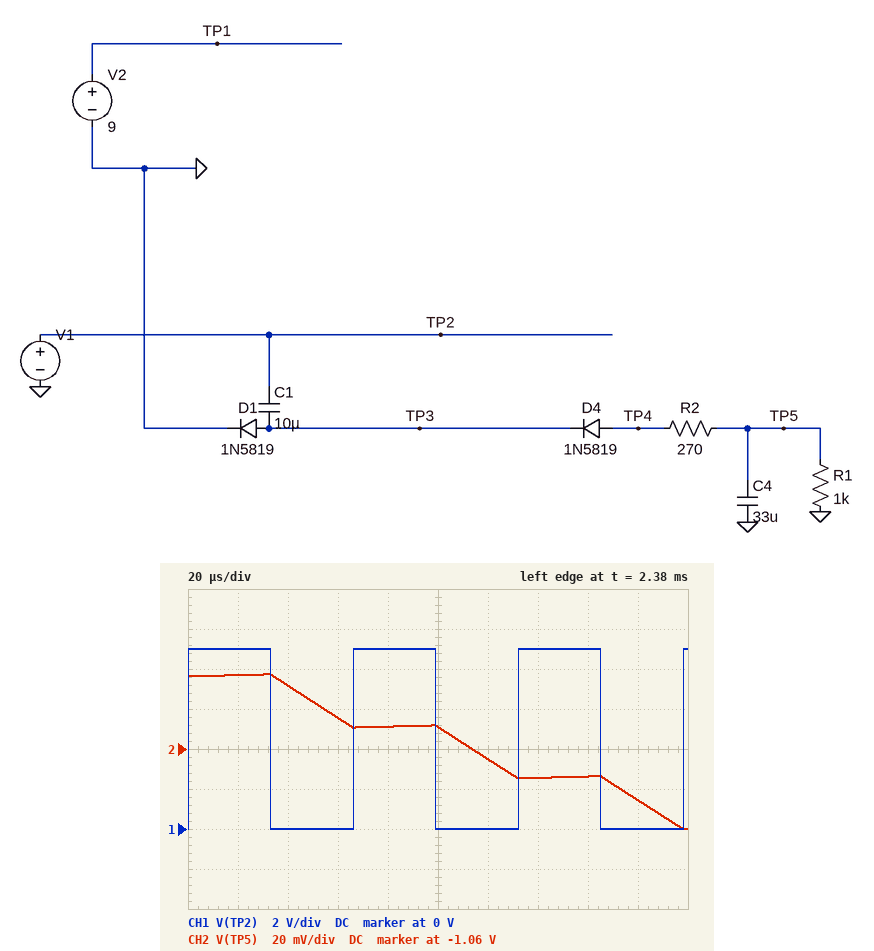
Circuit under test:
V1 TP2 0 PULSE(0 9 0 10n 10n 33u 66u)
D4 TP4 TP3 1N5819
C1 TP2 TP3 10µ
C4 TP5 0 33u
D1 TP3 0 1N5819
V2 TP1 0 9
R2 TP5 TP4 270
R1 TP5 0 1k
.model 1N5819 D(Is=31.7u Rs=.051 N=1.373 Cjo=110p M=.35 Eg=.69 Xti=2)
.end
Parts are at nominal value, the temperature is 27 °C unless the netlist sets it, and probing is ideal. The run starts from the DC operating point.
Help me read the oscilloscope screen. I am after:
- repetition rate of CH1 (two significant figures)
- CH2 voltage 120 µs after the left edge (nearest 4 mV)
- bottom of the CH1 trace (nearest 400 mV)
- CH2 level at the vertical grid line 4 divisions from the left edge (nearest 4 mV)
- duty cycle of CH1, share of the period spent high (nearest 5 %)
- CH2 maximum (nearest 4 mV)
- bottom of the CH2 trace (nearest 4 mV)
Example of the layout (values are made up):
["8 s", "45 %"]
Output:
["15 kHz", "-1.064 V", "0 V", "-1.048 V", "50 %", "-1.024 V", "-1.100 V"]
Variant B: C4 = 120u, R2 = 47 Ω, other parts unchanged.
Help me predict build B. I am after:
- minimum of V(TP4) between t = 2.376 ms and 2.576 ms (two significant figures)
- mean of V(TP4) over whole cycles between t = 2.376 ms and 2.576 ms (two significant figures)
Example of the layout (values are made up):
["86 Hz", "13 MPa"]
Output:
["-8.5 V", "-4.9 V"]
